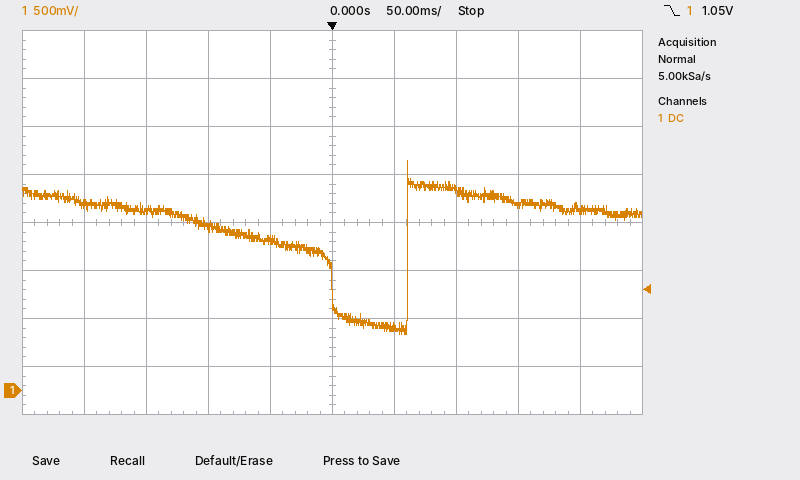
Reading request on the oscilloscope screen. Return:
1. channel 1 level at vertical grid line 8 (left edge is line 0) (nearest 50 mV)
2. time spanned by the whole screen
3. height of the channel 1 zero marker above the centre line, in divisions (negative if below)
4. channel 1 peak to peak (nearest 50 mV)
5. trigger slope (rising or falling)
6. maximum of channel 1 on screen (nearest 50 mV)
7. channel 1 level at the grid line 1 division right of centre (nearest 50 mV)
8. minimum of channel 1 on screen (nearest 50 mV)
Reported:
1.95 V
500 ms
-3.5 div
1.80 V
falling
2.40 V
650 mV
600 mV
